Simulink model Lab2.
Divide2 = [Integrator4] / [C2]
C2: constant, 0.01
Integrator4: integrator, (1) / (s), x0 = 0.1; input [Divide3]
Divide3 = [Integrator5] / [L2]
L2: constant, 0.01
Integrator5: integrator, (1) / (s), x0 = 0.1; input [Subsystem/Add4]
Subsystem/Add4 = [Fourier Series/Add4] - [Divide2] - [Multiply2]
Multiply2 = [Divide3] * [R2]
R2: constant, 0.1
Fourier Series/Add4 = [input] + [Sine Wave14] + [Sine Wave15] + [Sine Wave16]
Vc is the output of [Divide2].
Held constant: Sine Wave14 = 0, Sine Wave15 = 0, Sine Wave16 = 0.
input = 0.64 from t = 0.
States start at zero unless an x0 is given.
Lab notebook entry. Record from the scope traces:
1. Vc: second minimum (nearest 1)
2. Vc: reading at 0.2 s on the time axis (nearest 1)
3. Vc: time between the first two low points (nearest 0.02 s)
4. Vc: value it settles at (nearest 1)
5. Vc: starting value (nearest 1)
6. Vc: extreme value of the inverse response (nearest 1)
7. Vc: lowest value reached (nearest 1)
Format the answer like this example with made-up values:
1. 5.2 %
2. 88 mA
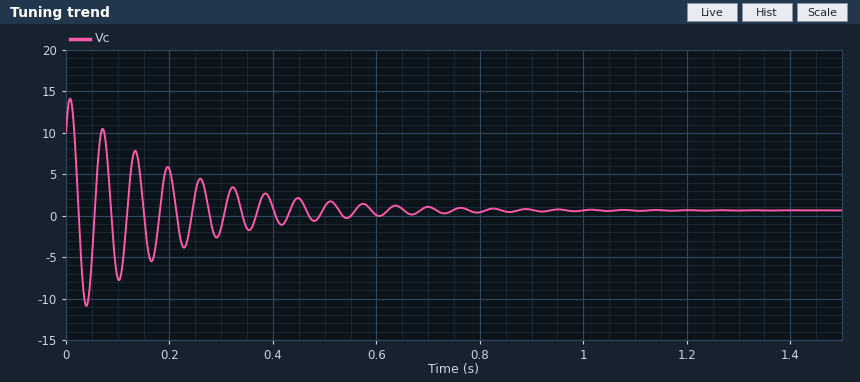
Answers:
1. -8
2. 6
3. 0.06 s
4. 1
5. 10
6. 14
7. -11
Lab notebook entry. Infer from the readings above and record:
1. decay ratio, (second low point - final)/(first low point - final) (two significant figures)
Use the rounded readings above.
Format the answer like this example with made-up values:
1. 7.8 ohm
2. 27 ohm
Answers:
1. 0.75
